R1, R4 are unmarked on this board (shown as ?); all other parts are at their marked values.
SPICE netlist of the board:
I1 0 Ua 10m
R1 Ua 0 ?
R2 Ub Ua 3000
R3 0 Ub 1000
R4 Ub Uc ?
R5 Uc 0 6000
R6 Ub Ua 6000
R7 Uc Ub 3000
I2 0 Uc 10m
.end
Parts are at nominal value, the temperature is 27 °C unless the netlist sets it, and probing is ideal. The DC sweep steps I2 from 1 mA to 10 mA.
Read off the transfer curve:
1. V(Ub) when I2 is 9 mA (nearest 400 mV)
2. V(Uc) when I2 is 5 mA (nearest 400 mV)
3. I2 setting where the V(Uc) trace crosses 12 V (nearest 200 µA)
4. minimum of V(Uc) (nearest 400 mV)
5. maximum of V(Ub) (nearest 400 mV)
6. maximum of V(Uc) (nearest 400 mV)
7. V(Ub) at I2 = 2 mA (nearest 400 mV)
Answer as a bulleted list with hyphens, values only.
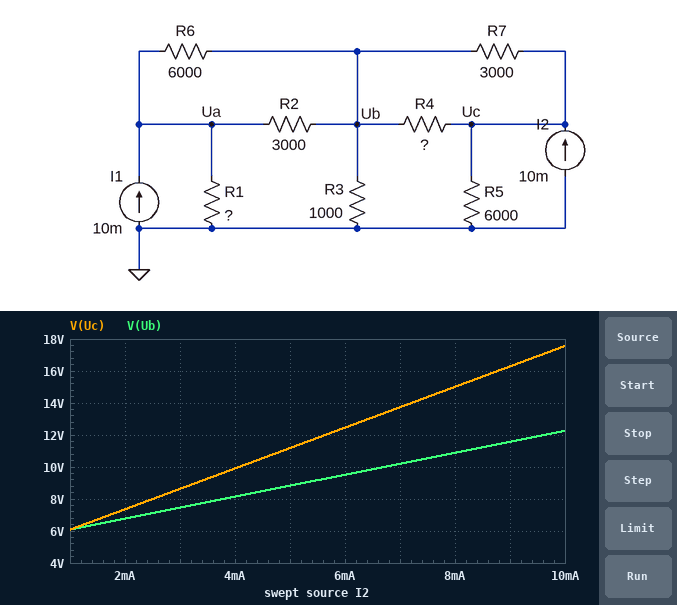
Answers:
- 11.6 V
- 11.2 V
- 5.6 mA
- 6.0 V
- 12.4 V
- 17.6 V
- 6.8 V
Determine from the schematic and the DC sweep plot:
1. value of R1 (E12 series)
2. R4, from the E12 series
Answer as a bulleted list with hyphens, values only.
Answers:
- 4.7 kΩ
- 1 kΩ
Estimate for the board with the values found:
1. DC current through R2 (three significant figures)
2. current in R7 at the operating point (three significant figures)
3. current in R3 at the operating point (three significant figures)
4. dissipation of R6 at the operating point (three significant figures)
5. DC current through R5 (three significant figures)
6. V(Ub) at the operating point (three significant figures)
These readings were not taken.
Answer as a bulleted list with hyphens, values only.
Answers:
- 3.46 mA
- 1.77 mA
- 12.3 mA
- 17.9 mW
- 2.93 mA
- 12.3 V
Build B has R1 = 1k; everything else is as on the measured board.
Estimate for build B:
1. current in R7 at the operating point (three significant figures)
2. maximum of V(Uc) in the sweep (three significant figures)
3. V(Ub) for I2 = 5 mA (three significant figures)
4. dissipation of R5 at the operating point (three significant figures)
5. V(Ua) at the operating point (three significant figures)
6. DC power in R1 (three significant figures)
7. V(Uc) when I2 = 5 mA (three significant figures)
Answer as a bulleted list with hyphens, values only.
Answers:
- 1.92 mA
- 14.0 V
- 5.25 V
- 32.7 mW
- 9.42 V
- 88.7 mW
- 8.00 V
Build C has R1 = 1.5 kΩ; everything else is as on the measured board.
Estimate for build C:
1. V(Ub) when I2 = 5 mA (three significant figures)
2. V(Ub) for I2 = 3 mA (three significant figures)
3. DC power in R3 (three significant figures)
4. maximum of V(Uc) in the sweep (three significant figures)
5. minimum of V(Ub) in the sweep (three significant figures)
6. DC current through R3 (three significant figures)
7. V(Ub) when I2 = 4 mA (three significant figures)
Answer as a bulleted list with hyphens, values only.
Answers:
- 6.09 V
- 4.85 V
- 84.4 mW
- 14.8 V
- 3.61 V
- 9.19 mA
- 5.47 V
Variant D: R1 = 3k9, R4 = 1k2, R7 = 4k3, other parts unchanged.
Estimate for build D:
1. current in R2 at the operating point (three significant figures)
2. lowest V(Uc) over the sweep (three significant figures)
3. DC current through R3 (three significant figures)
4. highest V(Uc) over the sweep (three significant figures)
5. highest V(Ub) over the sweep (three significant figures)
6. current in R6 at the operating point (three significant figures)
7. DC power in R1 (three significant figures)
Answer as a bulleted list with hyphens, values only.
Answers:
- 3.09 mA
- 5.73 V
- 11.6 mA
- 18.2 V
- 11.6 V
- 1.55 mA
- 112 mW
